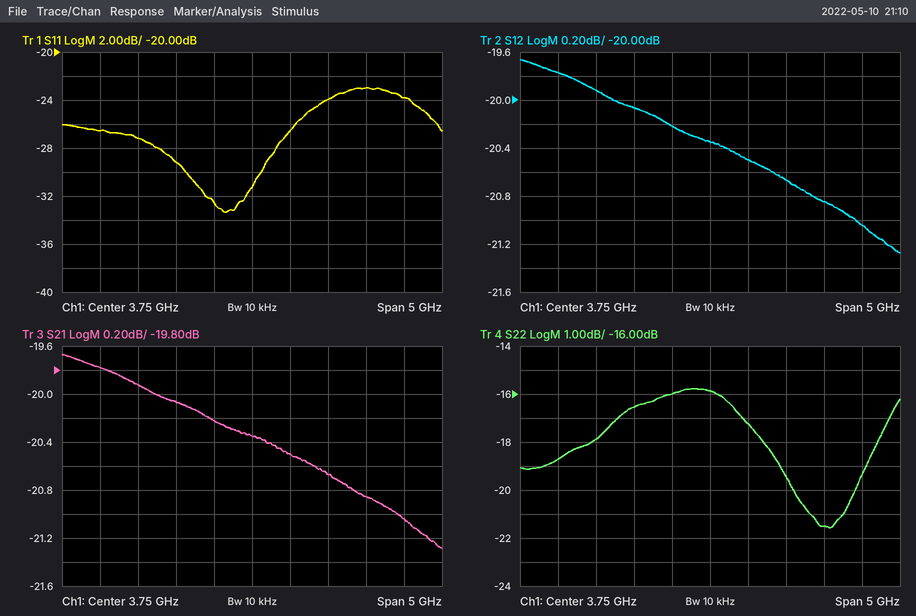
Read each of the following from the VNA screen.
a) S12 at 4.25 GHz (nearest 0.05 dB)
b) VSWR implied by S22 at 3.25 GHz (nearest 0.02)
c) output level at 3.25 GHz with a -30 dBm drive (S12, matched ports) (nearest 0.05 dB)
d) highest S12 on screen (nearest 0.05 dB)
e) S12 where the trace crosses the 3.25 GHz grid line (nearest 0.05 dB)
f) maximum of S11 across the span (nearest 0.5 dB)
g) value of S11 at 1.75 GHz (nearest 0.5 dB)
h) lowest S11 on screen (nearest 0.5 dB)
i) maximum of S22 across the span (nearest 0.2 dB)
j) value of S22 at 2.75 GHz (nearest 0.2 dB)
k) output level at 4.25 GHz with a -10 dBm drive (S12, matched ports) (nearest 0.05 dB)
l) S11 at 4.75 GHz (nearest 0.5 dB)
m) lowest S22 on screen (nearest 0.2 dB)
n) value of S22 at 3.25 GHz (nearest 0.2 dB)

-20.50 dB
1.38
-50.20 dBm
-19.65 dB
-20.20 dB
-23.0 dB
-26.5 dB
-33.5 dB
-15.8 dB
-16.6 dB
-30.50 dBm
-24.0 dB
-21.6 dB
-16.0 dB
